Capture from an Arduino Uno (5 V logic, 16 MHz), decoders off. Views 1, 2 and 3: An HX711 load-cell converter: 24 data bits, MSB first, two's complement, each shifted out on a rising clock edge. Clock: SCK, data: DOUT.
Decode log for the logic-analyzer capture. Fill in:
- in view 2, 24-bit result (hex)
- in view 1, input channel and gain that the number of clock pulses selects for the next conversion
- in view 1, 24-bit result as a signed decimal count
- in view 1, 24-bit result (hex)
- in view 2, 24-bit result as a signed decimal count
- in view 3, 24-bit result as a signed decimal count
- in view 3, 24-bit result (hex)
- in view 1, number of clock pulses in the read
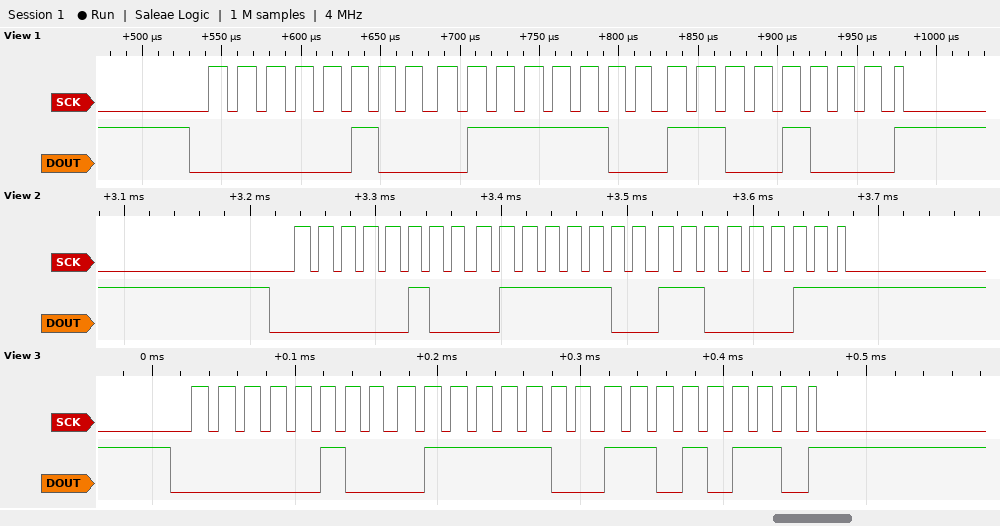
0x047CC3
channel A, gain 128
294088
0x047CC8
294083
294102
0x047CD6
25
